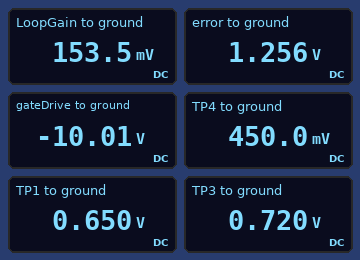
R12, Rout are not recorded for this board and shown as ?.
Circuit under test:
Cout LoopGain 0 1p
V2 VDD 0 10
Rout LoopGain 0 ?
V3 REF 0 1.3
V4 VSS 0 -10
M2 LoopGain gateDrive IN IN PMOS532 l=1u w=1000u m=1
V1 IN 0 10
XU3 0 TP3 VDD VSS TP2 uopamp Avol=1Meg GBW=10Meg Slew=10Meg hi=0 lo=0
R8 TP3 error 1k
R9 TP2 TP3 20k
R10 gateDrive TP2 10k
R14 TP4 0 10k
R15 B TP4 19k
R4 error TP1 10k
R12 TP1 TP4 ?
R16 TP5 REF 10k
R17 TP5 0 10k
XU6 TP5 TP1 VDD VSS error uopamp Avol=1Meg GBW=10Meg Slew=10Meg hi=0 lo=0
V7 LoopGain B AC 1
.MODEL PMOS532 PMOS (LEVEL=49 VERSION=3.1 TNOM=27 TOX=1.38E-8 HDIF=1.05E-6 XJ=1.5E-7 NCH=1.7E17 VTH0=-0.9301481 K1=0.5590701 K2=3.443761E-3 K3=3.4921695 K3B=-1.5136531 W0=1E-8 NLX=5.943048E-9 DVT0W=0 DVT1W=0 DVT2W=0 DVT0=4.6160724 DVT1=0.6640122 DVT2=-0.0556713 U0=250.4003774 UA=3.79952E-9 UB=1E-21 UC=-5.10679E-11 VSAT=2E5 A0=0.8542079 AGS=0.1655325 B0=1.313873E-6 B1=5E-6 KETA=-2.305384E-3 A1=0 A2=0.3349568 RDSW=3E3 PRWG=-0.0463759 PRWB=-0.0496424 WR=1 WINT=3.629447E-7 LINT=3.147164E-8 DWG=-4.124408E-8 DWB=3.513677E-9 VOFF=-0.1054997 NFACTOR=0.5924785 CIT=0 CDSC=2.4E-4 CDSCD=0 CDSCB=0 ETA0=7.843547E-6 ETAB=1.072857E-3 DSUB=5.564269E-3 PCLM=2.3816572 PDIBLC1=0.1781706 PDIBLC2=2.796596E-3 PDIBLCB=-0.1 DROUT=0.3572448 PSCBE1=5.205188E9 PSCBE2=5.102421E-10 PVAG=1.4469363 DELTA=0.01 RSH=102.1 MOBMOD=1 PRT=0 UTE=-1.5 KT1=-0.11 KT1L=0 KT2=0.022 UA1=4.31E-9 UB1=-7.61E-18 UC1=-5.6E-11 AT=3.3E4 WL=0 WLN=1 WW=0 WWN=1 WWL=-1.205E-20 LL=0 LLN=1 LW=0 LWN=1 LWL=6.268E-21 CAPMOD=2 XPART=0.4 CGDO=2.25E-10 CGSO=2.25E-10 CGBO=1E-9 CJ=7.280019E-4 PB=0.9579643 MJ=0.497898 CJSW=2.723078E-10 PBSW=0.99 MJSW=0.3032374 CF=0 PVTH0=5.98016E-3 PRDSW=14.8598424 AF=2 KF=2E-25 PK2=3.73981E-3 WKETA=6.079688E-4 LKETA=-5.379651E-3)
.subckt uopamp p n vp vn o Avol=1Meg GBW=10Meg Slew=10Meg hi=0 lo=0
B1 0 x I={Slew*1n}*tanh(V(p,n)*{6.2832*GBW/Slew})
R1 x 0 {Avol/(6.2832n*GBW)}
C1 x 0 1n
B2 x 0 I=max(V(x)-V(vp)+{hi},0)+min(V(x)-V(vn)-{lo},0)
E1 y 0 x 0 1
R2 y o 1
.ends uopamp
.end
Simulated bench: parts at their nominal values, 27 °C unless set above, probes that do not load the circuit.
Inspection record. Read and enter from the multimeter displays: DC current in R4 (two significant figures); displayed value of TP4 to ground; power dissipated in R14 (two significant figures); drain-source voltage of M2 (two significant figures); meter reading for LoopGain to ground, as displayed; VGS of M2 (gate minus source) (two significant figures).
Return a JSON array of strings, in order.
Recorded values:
["61 µA", "450.0 mV", "20 µW", "-9.8 V", "153.5 mV", "-20 V"]
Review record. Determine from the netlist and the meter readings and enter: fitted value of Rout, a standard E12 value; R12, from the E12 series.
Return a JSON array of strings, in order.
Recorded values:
["3.3 Ω", "3.3 kΩ"]
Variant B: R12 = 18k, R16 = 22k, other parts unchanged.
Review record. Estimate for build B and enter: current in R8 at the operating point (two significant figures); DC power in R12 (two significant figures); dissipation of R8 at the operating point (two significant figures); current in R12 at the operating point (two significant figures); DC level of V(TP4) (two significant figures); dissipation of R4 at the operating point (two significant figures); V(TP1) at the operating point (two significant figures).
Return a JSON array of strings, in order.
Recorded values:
["500 µA", "3.7 µW", "250 µW", "14 µA", "150 mV", "2.1 µW", "410 mV"]
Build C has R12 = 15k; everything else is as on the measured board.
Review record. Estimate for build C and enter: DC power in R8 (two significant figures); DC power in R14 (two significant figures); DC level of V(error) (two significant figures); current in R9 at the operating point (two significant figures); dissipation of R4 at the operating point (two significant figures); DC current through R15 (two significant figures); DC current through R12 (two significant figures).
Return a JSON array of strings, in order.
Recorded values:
["270 µW", "5.5 µW", "930 mV", "520 µA", "7.7 µW", "4.3 µA", "28 µA"]
